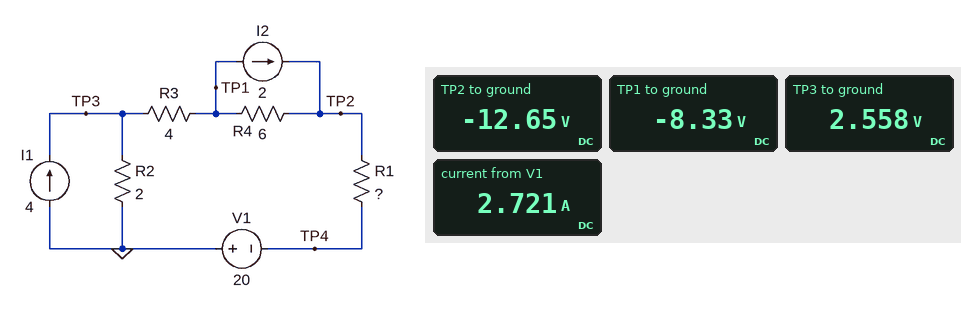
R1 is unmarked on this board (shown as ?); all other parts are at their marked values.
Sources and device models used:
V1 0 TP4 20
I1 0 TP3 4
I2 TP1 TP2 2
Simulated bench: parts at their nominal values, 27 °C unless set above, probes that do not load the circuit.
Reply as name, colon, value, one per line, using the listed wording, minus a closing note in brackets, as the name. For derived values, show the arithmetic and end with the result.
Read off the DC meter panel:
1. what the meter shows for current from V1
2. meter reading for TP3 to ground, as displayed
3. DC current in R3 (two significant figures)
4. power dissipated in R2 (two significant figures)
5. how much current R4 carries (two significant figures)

what the meter shows for current from V1: 2.721 A
meter reading for TP3 to ground, as displayed: 2.558 V
DC current in R3: (2.558 V - (-8.33 V)) / 4 Ω = 2.7 A
power dissipated in R2: (2.558 V)^2 / 2 Ω = 3.3 W
how much current R4 carries: (-8.33 V - (-12.65 V)) / 6 Ω = 720 mA
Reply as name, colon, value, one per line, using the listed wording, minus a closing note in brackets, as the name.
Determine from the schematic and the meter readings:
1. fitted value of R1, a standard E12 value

fitted value of R1, a standard E12 value: 2.7 Ω
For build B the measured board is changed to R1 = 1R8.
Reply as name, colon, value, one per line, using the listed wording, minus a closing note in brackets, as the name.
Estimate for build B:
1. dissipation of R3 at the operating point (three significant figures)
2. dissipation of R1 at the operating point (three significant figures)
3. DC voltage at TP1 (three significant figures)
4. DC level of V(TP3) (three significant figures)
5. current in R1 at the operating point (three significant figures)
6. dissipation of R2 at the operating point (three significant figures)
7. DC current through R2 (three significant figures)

dissipation of R3 at the operating point: 33.6 W
dissipation of R1 at the operating point: 15.1 W
DC voltage at TP1: -9.39 V
DC level of V(TP3): 2.20 V
current in R1 at the operating point: 2.90 A
dissipation of R2 at the operating point: 2.43 W
DC current through R2: 1.10 A
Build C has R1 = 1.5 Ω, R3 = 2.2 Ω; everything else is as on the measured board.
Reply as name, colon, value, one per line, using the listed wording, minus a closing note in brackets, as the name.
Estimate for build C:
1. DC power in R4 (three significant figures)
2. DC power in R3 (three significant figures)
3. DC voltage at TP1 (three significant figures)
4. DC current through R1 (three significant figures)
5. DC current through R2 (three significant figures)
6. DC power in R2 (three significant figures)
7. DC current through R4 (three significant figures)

DC power in R4: 12.1 W
DC power in R3: 25.7 W
DC voltage at TP1: -6.36 V
DC current through R1: 3.42 A
DC current through R2: 581 mA
DC power in R2: 676 mW
DC current through R4: 1.42 A
